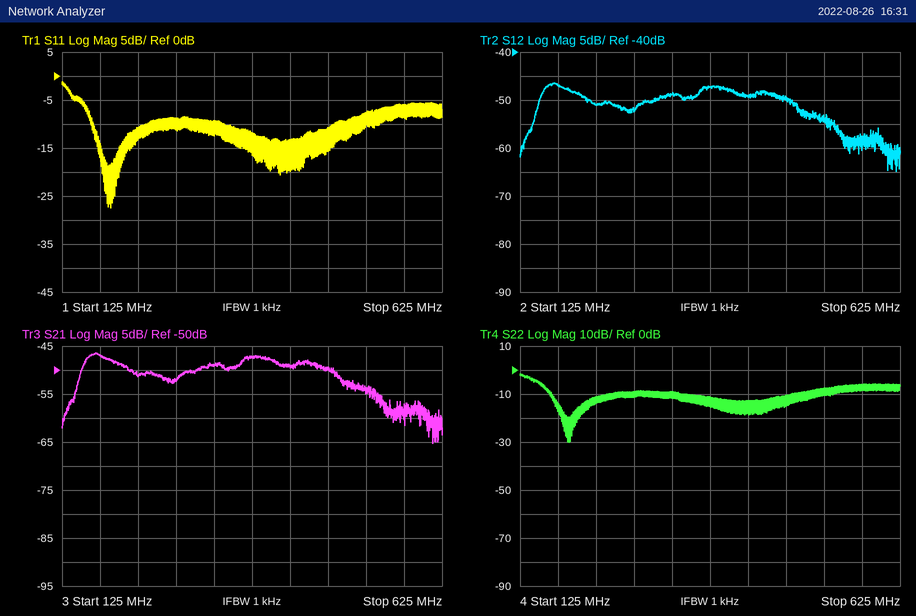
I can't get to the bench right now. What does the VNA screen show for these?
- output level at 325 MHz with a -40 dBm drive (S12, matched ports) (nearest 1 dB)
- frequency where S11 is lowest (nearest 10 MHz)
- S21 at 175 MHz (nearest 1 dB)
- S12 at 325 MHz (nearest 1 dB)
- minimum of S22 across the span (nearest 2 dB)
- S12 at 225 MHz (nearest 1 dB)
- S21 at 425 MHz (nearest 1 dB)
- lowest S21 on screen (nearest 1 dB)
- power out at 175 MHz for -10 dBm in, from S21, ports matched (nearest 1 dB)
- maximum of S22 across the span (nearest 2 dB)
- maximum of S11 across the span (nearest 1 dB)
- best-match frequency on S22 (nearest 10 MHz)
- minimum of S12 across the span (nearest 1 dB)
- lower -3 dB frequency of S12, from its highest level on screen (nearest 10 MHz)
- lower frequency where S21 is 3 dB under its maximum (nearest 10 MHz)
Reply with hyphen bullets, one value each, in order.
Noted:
- -89 dBm
- 190 MHz
- -47 dB
- -49 dB
- -30 dB
- -51 dB
- -49 dB
- -65 dB
- -57 dBm
- -2 dB
- -1 dB
- 190 MHz
- -65 dB
- 150 MHz
- 150 MHz
